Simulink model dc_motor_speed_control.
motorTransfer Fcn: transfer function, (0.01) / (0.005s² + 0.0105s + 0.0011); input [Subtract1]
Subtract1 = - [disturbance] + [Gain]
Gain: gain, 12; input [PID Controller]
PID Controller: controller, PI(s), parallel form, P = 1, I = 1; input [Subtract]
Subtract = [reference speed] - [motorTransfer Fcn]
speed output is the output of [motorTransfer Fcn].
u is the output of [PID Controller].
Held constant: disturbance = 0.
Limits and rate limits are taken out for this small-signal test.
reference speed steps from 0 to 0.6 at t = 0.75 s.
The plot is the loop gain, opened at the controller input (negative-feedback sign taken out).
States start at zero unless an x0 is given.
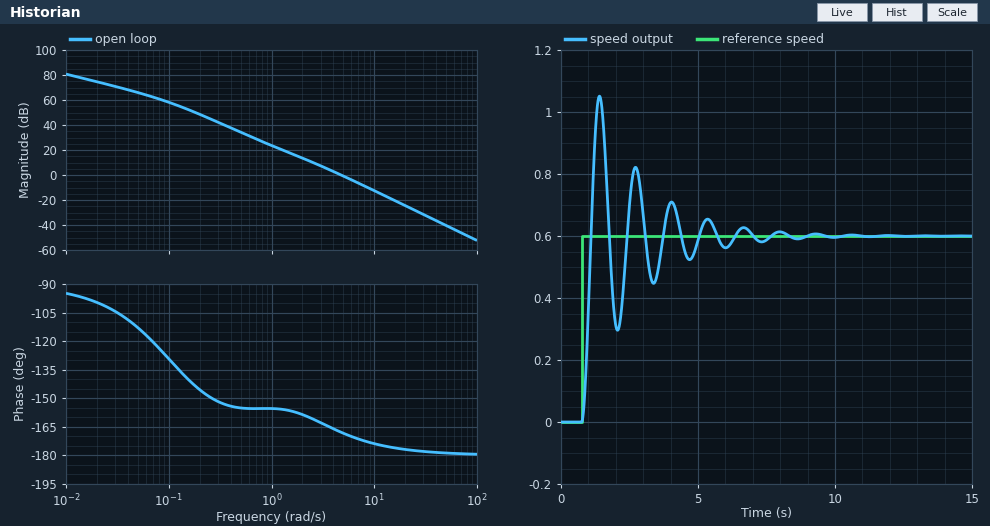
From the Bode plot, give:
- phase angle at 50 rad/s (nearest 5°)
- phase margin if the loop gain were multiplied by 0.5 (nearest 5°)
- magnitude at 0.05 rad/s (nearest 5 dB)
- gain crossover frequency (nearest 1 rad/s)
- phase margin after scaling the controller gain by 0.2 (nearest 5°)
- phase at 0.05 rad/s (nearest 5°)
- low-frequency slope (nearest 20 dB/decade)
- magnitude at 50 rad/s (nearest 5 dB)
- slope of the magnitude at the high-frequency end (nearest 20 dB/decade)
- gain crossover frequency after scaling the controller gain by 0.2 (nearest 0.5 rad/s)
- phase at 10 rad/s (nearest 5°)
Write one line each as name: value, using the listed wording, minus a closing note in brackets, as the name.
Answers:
phase angle at 50 rad/s: -180°
phase margin if the loop gain were multiplied by 0.5: 15°
magnitude at 0.05 rad/s: 65 dB
gain crossover frequency: 5 rad/s
phase margin after scaling the controller gain by 0.2: 20°
phase at 0.05 rad/s: -115°
low-frequency slope: -20 dB/decade
magnitude at 50 rad/s: -40 dB
slope of the magnitude at the high-frequency end: -40 dB/decade
gain crossover frequency after scaling the controller gain by 0.2: 2.0 rad/s
phase at 10 rad/s: -175°
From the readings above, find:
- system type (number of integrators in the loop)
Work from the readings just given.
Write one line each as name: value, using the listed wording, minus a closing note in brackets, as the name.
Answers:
system type: 1
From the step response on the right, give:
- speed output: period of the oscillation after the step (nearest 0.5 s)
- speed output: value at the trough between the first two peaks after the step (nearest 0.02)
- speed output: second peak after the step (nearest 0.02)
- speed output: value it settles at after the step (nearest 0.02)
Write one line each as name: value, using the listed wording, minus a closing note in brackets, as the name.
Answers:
speed output: period of the oscillation after the step: 1.5 s
speed output: value at the trough between the first two peaks after the step: 0.30
speed output: second peak after the step: 0.82
speed output: value it settles at after the step: 0.60
